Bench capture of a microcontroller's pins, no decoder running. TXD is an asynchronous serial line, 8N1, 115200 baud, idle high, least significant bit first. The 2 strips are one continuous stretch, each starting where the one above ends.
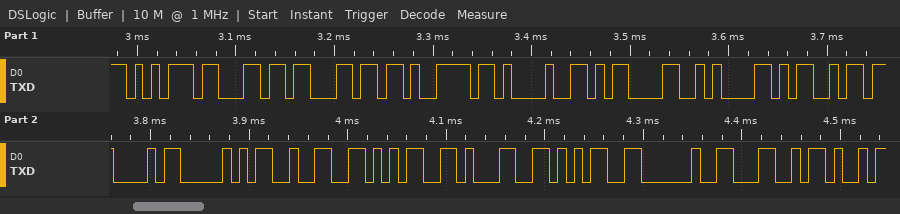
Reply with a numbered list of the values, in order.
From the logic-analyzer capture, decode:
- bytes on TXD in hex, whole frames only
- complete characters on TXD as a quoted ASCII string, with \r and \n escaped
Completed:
1. 75 6C 6C 79 21 0D 0A 4D 43 50 32 35 31 35 20 4C
2. "ully!\r\nMCP2515 L"
